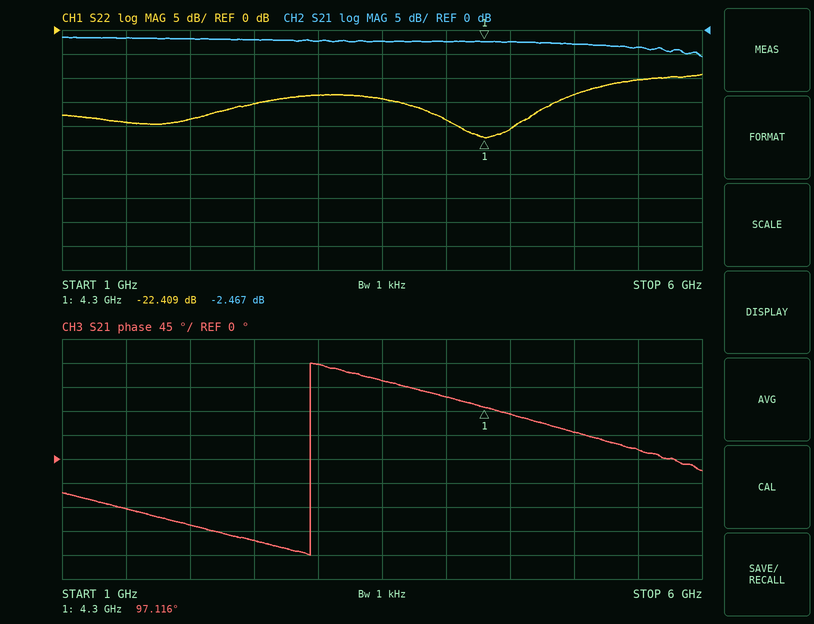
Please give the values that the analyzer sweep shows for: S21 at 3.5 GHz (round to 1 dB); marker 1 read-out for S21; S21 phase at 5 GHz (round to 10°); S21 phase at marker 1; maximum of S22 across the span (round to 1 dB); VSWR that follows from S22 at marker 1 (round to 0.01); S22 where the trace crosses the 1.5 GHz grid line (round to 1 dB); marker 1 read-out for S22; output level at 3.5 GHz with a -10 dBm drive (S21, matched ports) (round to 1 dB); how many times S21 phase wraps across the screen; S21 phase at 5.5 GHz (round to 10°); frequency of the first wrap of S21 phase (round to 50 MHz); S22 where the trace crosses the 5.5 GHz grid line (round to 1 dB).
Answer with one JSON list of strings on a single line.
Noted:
["-2 dB", "-2.467 dB", "50°", "97.116°", "-9 dB", "1.16", "-19 dB", "-22.409 dB", "-12 dBm", "1", "20°", "2.95 GHz", "-10 dB"]
